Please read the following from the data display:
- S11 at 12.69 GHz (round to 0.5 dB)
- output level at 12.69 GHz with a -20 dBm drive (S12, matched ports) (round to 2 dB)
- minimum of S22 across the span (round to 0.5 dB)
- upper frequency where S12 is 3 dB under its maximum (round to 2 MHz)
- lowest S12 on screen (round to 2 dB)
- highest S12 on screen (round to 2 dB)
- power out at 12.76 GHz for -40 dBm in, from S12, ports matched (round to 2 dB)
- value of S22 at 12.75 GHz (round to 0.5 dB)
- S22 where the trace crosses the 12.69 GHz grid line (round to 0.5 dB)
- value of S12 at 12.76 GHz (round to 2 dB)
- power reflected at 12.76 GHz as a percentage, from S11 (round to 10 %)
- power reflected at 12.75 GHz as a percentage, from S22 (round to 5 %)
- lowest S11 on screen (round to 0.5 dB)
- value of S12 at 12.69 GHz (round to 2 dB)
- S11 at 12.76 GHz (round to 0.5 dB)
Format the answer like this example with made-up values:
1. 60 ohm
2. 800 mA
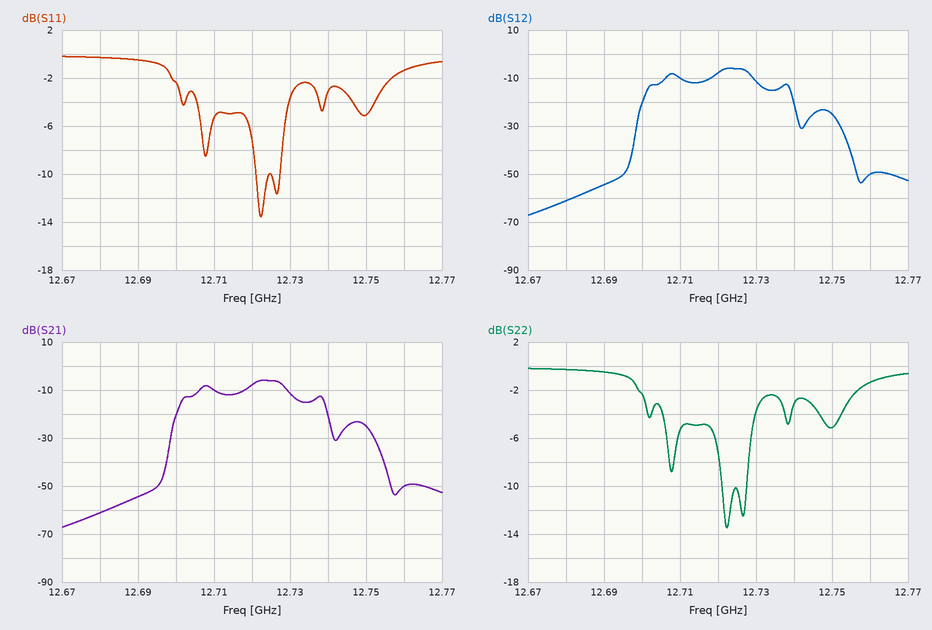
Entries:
1. -0.5 dB
2. -74 dBm
3. -13.5 dB
4. 12.728 GHz
5. -68 dB
6. -6 dB
7. -90 dBm
8. -5.0 dB
9. -0.5 dB
10. -50 dB
11. 70 %
12. 30 %
13. -13.5 dB
14. -54 dB
15. -1.5 dB
